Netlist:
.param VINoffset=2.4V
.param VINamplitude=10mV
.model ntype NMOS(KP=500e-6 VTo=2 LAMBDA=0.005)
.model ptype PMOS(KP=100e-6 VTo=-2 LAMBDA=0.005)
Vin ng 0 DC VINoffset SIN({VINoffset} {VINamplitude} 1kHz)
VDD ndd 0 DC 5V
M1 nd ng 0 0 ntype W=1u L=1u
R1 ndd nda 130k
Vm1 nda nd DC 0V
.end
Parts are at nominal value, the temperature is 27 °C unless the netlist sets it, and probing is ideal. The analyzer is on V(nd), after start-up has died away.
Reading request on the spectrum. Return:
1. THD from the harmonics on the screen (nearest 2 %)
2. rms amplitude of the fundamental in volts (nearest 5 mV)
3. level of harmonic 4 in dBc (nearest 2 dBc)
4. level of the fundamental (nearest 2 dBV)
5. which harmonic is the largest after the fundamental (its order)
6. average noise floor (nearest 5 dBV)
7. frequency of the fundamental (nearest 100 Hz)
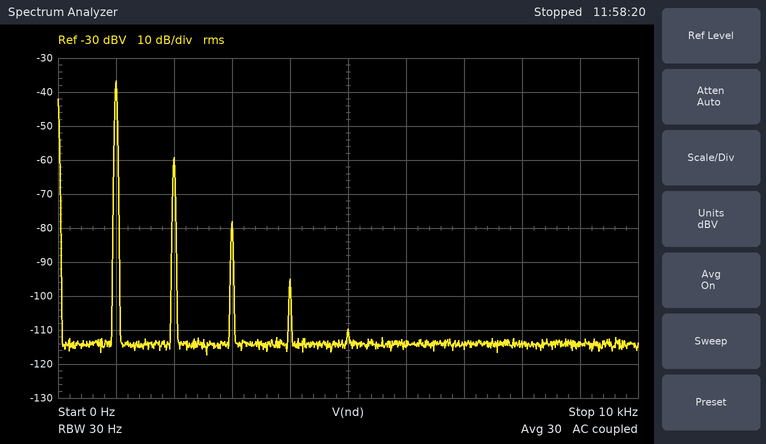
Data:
8 %
15 mV
-58 dBc
-36 dBV
2
-115 dBV
1.0 kHz
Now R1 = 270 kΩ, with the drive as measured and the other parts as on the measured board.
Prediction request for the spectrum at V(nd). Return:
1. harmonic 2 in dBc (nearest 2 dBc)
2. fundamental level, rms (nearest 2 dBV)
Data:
-34 dBc
-52 dBV
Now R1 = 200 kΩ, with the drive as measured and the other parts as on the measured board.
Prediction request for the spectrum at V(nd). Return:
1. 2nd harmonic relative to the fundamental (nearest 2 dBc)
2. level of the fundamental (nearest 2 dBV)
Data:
-32 dBc
-48 dBV
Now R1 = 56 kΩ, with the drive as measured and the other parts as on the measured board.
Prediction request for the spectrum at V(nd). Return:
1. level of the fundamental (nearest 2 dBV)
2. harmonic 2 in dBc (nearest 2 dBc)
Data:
-22 dBV
-44 dBc
